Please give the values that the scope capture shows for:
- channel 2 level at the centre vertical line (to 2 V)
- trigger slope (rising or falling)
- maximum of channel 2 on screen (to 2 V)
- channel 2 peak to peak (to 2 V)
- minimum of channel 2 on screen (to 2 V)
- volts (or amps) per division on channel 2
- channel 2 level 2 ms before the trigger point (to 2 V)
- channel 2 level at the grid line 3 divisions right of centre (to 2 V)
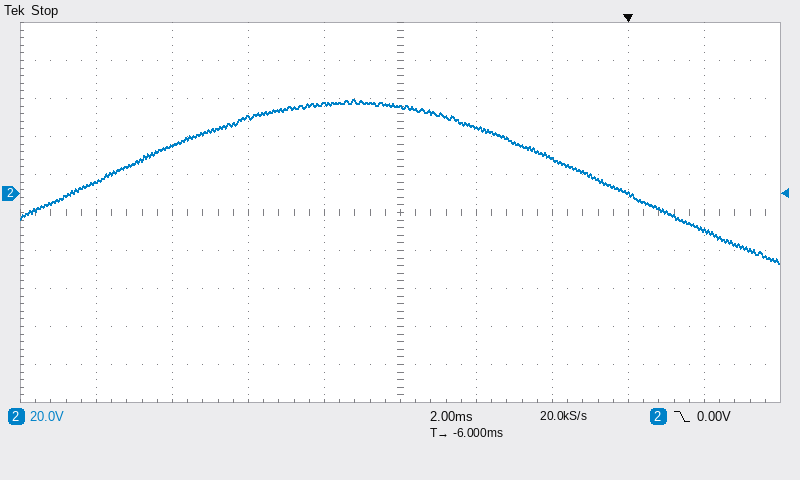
46 V
falling
50 V
86 V
-36 V
20 V
18 V
0 V
